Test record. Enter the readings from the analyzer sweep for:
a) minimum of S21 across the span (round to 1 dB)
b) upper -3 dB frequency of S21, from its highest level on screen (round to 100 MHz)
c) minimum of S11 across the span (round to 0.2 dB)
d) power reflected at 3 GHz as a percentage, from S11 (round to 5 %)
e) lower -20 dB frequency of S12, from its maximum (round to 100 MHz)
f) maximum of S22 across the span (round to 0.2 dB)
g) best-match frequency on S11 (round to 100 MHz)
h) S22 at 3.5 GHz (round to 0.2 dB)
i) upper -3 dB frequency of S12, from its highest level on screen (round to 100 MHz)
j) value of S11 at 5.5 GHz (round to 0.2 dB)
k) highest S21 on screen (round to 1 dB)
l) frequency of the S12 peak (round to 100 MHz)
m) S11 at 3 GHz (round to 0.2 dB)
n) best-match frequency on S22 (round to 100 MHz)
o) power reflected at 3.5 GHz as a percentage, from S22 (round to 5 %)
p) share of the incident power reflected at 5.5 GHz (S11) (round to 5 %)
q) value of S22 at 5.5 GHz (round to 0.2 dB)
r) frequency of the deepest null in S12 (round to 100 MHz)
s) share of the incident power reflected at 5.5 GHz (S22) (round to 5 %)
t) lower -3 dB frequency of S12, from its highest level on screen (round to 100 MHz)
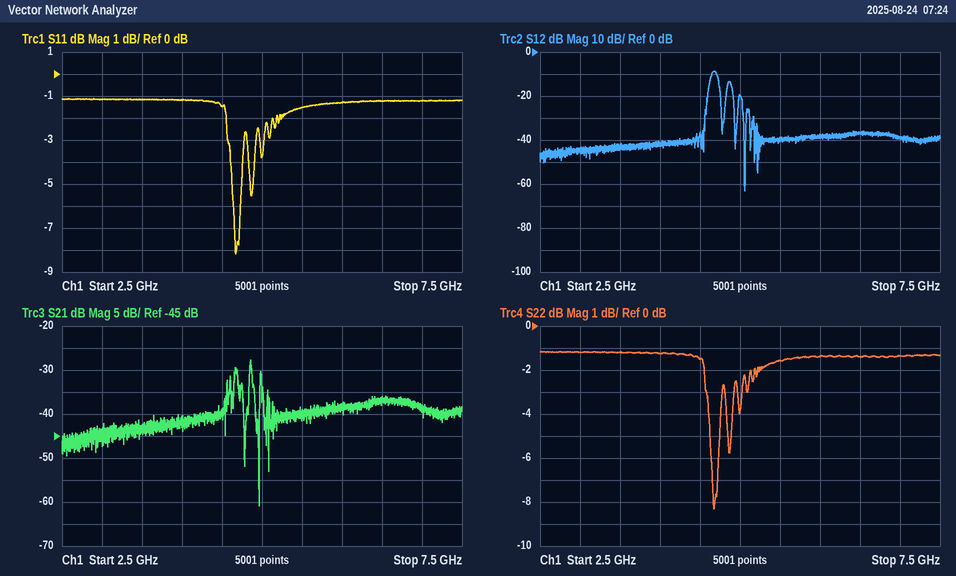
-61 dB
4.9 GHz
-8.2 dB
75 %
4.6 GHz
-1.2 dB
4.7 GHz
-1.2 dB
4.7 GHz
-1.6 dB
-28 dB
4.7 GHz
-1.2 dB
4.7 GHz
75 %
70 %
-1.6 dB
5.1 GHz
70 %
4.6 GHz
